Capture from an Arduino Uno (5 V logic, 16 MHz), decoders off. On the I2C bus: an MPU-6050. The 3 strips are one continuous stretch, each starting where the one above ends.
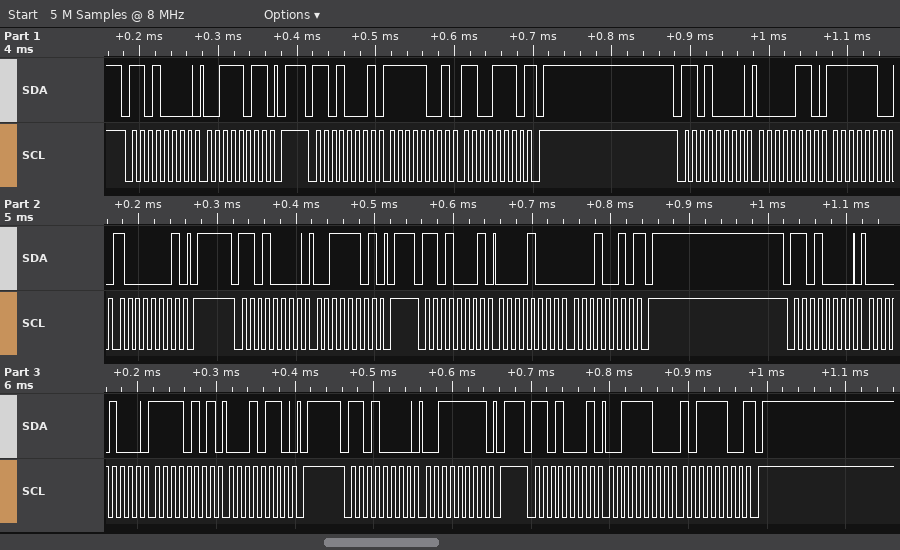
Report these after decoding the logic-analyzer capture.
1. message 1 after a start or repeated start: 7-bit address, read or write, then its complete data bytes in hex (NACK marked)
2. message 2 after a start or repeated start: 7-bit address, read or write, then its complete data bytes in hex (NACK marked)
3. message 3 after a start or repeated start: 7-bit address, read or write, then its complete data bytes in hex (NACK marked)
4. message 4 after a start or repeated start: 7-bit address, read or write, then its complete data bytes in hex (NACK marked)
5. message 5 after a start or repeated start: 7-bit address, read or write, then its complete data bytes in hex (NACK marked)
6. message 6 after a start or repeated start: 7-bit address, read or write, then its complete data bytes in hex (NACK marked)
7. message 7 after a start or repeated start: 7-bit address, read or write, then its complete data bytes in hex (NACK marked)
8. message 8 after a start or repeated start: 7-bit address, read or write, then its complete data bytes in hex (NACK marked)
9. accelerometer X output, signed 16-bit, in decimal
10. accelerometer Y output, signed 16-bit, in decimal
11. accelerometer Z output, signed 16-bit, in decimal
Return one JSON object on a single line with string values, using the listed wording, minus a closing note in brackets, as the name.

{"message 1 after a start or repeated start: 7-bit address, read or write, then its complete data bytes in hex": "0x68 write: 3B", "message 2 after a start or repeated start: 7-bit address, read or write, then its complete data bytes in hex": "0x68 read: F9 CE NACK", "message 3 after a start or repeated start: 7-bit address, read or write, then its complete data bytes in hex": "0x68 write: 06 FC 81", "message 4 after a start or repeated start: 7-bit address, read or write, then its complete data bytes in hex": "0x68 write: 3D", "message 5 after a start or repeated start: 7-bit address, read or write, then its complete data bytes in hex": "0x68 read: 08 12 NACK", "message 6 after a start or repeated start: 7-bit address, read or write, then its complete data bytes in hex": "0x68 write: 08 F5 16", "message 7 after a start or repeated start: 7-bit address, read or write, then its complete data bytes in hex": "0x68 write: 3F", "message 8 after a start or repeated start: 7-bit address, read or write, then its complete data bytes in hex": "0x68 read: 3C BC NACK", "accelerometer X output, signed 16-bit, in decimal": "-1586", "accelerometer Y output, signed 16-bit, in decimal": "2066", "accelerometer Z output, signed 16-bit, in decimal": "15548"}
